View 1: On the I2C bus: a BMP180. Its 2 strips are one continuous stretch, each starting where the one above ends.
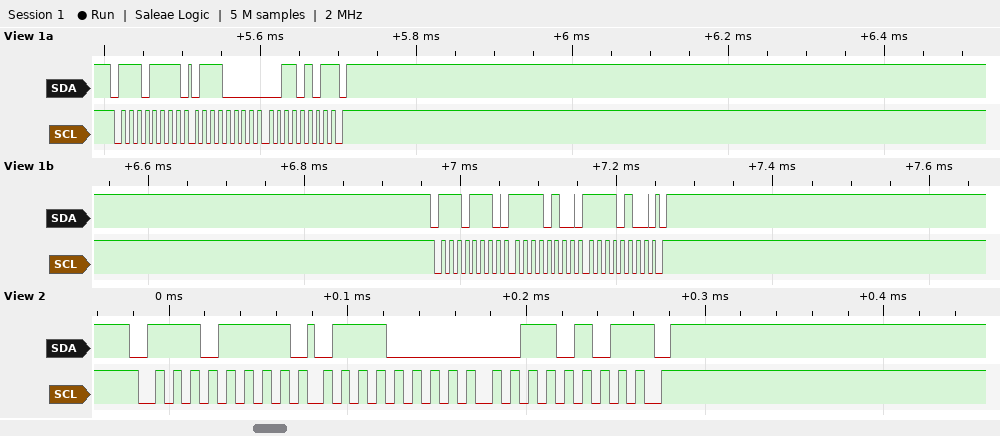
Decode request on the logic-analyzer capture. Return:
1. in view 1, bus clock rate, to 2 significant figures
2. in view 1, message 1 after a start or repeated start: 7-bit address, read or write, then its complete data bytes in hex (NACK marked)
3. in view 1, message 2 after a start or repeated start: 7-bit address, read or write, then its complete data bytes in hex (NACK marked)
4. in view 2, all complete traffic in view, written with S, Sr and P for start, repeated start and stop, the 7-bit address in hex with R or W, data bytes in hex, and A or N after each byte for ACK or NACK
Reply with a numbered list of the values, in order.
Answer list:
1. 100 kHz
2. 0x77 read: 70 35 NACK
3. 0x77 write: F4 F4
4. S 77R A 70 A 35 N P
